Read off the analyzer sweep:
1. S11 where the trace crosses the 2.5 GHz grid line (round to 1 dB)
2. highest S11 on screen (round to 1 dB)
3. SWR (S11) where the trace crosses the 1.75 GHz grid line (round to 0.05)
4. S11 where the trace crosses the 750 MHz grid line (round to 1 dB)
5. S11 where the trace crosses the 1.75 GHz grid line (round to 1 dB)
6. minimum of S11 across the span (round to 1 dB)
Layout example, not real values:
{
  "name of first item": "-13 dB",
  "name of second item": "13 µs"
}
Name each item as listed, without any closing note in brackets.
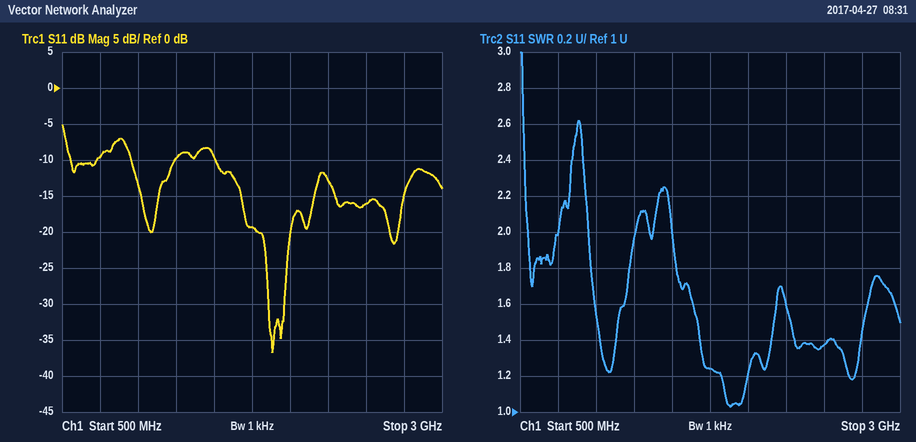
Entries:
{
  "S11 where the trace crosses the 2.5 GHz grid line": "-16 dB",
  "highest S11 on screen": "-5 dB",
  "SWR (S11) where the trace crosses the 1.75 GHz grid line": "1.25",
  "S11 where the trace crosses the 750 MHz grid line": "-10 dB",
  "S11 where the trace crosses the 1.75 GHz grid line": "-19 dB",
  "minimum of S11 across the span": "-37 dB"
}
